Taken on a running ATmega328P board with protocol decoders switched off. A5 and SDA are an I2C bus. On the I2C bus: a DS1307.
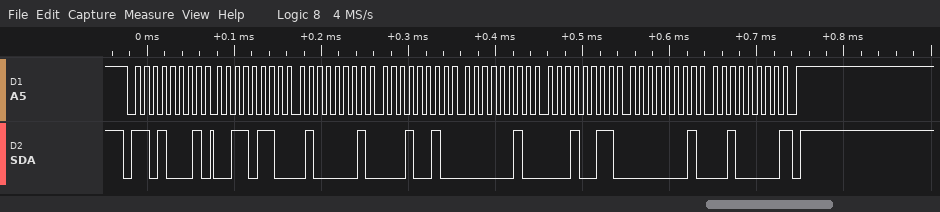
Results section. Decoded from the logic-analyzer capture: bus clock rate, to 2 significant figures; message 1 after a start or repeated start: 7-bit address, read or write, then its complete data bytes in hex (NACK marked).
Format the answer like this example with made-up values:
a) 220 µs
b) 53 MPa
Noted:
a) 100 kHz
b) 0x68 read: 36 41 12 02 13 01 20 NACK
